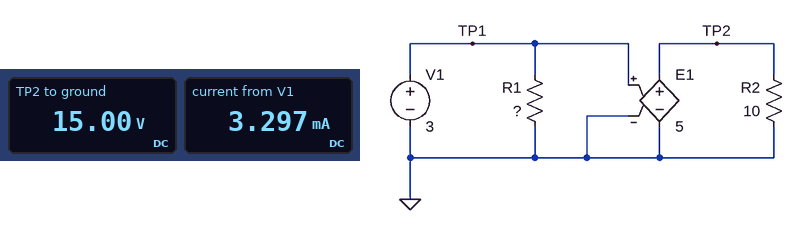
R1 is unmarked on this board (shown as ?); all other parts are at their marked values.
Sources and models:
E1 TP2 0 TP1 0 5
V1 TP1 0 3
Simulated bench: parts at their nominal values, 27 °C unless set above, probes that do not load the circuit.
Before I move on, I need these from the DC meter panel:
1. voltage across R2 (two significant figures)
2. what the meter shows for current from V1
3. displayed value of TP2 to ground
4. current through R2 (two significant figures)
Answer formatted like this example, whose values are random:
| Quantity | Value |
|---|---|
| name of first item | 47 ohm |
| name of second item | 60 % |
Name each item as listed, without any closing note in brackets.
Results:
| Quantity | Value |
|---|---|
| voltage across R2 | 15 V |
| what the meter shows for current from V1 | 3.297 mA |
| displayed value of TP2 to ground | 15.00 V |
| current through R2 | 1.5 A |
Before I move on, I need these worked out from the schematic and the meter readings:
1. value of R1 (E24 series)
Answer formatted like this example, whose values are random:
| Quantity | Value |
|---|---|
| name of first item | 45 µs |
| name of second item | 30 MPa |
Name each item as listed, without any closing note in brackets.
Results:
| Quantity | Value |
|---|---|
| value of R1 | 910 Ω |
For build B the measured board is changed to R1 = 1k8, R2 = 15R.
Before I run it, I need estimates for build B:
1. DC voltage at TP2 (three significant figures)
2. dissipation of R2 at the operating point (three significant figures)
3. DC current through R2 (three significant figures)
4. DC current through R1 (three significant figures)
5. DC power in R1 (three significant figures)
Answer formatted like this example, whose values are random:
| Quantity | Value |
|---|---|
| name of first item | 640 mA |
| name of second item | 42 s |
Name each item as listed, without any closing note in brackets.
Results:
| Quantity | Value |
|---|---|
| DC voltage at TP2 | 15.0 V |
| dissipation of R2 at the operating point | 15.0 W |
| DC current through R2 | 1.00 A |
| DC current through R1 | 1.67 mA |
| DC power in R1 | 5.00 mW |
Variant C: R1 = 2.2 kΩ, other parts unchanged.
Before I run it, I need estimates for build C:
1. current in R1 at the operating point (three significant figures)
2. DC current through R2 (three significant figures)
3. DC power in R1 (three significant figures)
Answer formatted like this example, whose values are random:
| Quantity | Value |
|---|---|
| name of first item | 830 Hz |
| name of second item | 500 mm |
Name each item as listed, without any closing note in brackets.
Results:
| Quantity | Value |
|---|---|
| current in R1 at the operating point | 1.36 mA |
| DC current through R2 | 1.50 A |
| DC power in R1 | 4.09 mW |
